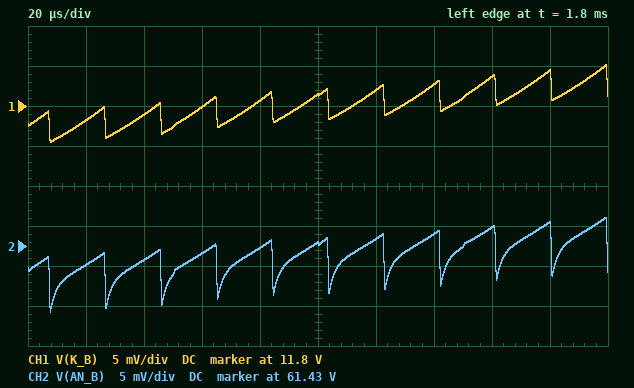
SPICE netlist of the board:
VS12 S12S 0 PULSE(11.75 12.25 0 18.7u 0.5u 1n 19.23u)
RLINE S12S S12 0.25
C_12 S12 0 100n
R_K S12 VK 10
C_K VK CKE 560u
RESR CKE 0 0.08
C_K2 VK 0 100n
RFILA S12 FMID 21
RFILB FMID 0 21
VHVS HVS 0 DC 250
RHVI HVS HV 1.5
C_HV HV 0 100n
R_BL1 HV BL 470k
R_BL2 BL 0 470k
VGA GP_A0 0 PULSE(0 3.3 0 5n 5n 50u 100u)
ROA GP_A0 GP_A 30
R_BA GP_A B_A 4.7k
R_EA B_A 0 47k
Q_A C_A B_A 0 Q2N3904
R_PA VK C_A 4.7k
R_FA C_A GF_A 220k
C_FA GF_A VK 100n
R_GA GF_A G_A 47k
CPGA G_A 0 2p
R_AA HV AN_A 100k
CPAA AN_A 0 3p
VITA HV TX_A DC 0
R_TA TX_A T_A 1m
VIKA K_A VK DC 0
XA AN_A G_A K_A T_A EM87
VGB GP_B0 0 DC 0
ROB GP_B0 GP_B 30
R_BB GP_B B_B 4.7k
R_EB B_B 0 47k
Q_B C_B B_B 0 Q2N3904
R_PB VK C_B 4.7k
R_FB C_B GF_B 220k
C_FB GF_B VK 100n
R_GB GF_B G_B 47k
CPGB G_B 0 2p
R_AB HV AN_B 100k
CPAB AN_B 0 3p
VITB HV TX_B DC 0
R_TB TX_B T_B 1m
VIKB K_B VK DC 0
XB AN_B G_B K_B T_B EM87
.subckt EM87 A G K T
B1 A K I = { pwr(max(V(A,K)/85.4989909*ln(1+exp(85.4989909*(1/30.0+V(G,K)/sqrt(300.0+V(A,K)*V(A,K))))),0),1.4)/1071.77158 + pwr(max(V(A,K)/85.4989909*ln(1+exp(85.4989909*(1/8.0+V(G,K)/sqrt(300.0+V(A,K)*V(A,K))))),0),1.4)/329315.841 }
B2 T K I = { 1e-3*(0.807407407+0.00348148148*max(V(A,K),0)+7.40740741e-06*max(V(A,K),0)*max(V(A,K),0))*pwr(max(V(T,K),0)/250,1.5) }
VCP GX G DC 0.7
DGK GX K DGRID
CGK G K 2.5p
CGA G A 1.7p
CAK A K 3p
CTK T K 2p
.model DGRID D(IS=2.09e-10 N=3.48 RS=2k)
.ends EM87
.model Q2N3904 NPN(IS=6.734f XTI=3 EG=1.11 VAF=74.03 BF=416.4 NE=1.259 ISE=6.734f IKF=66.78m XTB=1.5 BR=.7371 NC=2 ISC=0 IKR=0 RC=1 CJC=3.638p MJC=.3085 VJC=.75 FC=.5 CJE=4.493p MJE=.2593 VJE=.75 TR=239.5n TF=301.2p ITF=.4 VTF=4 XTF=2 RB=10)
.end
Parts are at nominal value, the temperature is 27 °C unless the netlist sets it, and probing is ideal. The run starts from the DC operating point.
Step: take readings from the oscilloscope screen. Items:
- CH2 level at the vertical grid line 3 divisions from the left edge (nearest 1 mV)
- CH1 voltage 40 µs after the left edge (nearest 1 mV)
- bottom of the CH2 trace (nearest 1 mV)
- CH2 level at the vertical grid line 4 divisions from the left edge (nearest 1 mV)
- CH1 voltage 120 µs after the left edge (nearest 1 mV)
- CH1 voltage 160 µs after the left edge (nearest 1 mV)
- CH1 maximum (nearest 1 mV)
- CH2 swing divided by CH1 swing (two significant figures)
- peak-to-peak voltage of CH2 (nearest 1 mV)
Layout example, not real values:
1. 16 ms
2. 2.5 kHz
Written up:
1. 61.429 V
2. 11.804 V
3. 61.422 V
4. 61.430 V
5. 11.807 V
6. 11.809 V
7. 11.810 V
8. 1.2
9. 12 mV
